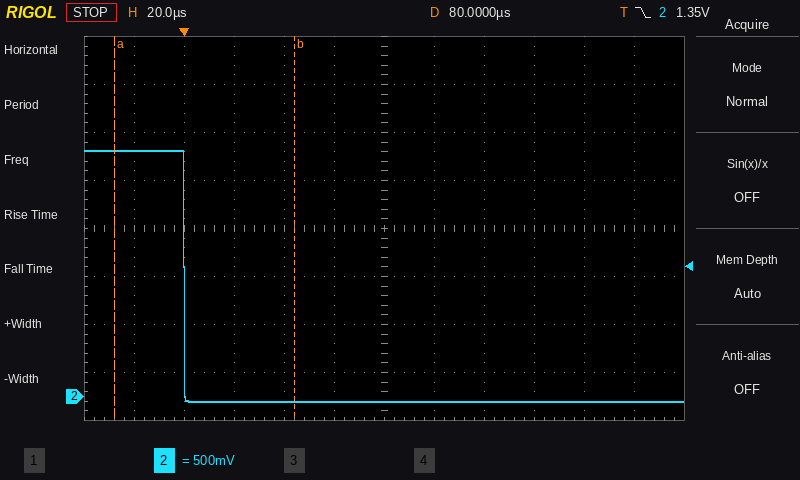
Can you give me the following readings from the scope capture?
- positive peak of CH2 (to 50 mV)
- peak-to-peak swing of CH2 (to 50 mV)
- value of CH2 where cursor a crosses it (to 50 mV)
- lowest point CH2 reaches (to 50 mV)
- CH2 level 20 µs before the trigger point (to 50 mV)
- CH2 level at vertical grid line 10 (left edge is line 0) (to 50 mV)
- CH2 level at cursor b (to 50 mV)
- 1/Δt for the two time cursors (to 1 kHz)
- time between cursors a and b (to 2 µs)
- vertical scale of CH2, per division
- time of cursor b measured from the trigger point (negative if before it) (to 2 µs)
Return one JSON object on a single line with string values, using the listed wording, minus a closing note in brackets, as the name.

{"positive peak of CH2": "2.55 V", "peak-to-peak swing of CH2": "2.60 V", "value of CH2 where cursor a crosses it": "2.55 V", "lowest point CH2 reaches": "-50 mV", "CH2 level 20 µs before the trigger point": "2.55 V", "CH2 level at vertical grid line 10 (left edge is line 0)": "-50 mV", "CH2 level at cursor b": "-50 mV", "1/Δt for the two time cursors": "14 kHz", "time between cursors a and b": "72 µs", "vertical scale of CH2, per division": "500 mV", "time of cursor b measured from the trigger point (negative if before it)": "+44 µs"}
